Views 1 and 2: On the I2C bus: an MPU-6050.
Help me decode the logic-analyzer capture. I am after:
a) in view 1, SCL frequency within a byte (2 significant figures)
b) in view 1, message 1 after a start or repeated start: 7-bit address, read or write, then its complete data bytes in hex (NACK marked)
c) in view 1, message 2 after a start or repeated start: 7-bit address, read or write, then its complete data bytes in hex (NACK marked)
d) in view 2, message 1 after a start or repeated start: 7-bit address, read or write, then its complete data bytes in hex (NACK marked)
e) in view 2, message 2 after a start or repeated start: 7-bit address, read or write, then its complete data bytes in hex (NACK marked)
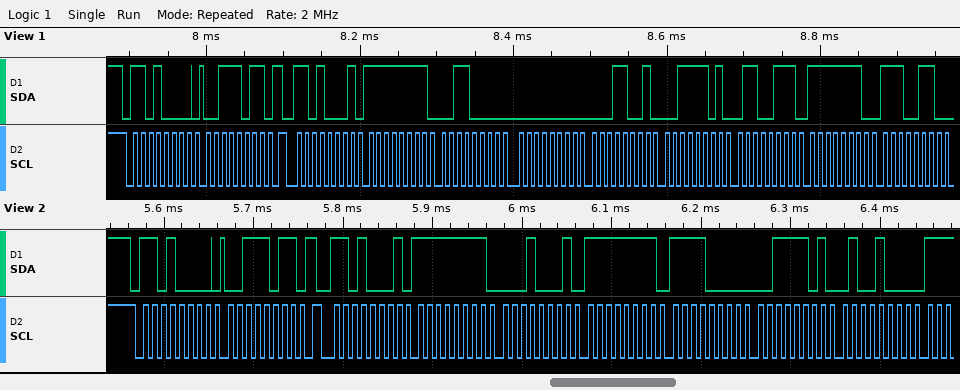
100 kHz
0x68 write: 3B
0x68 read: FF 30 00 19 3D 67 FE E6
0x68 write: 3B
0x68 read: FF 11 FF F0 3D 48
